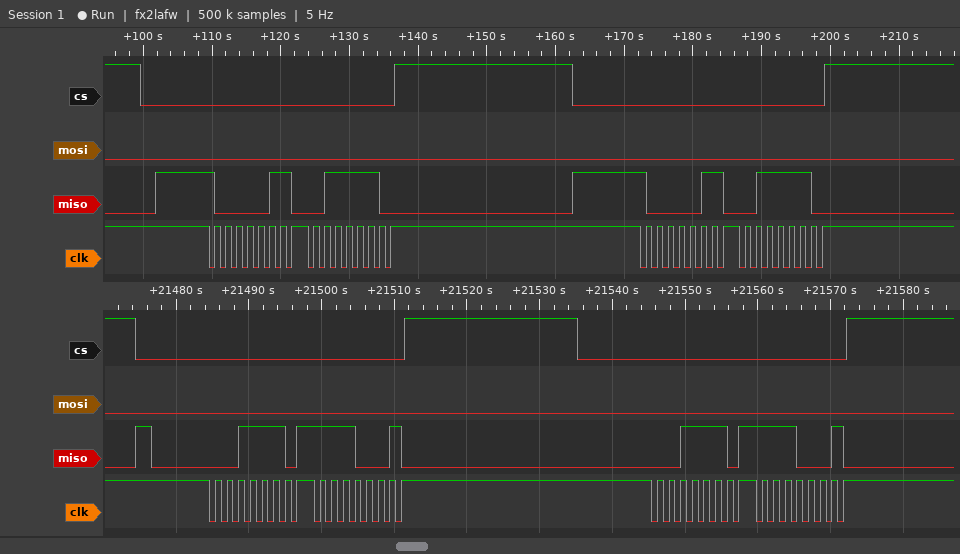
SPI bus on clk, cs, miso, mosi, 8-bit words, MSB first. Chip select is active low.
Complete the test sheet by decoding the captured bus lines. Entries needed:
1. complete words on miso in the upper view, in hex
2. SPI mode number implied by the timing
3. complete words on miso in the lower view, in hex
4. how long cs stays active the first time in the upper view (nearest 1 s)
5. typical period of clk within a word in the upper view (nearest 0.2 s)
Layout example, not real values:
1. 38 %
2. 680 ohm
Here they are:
1. 83, 3E, 83, 3E
2. 2
3. 1E, F1, 1E, F1
4. 37 s
5. 1.6 s
